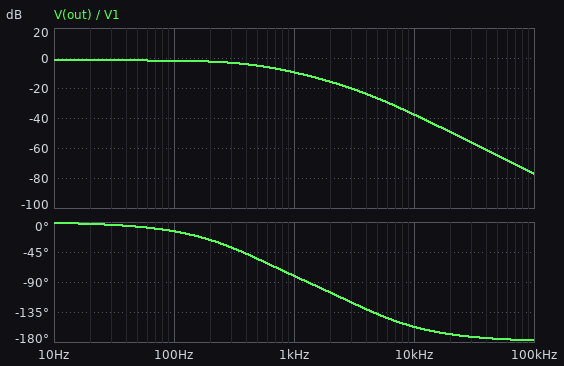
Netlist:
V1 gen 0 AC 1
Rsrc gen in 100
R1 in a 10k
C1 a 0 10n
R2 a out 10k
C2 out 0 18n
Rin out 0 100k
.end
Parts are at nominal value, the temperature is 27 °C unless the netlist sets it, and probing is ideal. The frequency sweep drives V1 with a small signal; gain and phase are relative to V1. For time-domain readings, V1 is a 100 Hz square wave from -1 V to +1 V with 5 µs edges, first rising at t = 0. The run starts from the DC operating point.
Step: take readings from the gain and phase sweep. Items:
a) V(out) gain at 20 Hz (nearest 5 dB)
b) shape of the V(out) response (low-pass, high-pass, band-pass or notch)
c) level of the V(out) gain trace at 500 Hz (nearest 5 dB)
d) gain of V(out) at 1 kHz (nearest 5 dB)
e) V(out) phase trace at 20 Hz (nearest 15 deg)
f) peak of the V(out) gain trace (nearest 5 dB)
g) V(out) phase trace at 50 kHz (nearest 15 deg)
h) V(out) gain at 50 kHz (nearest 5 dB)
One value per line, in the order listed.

0 dB
low-pass
-5 dB
-10 dB
0 deg
0 dB
-180 deg
-65 dB
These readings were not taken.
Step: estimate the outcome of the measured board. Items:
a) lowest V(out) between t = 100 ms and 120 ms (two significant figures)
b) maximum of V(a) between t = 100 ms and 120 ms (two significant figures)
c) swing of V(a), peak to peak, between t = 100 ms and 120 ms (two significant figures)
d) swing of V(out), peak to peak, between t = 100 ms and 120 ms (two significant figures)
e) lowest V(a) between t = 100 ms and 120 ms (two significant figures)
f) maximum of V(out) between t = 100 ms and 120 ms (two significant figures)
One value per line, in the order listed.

-830 mV
920 mV
1.8 V
1.7 V
-920 mV
830 mV
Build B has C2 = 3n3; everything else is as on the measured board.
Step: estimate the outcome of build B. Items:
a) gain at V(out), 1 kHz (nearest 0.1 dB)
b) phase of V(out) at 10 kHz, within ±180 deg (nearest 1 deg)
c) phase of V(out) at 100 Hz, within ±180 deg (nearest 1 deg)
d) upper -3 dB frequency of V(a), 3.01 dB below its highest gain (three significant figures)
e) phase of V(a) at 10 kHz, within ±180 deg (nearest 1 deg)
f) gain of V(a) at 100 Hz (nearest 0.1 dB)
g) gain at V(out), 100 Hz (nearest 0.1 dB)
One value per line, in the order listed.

-3.8 dB
-137 deg
-5 deg
1.30 kHz
-75 deg
-0.8 dB
-1.6 dB
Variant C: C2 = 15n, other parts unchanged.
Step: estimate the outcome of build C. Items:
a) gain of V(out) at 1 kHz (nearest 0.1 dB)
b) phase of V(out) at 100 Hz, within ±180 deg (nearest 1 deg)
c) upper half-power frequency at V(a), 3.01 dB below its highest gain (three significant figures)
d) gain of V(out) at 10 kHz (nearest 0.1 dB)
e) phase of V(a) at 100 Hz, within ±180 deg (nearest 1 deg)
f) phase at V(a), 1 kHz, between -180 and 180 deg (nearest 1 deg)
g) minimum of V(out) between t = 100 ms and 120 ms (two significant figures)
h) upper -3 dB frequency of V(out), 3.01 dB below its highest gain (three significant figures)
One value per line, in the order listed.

-8.5 dB
-12 deg
659 Hz
-36.1 dB
-7 deg
-36 deg
-830 mV
518 Hz
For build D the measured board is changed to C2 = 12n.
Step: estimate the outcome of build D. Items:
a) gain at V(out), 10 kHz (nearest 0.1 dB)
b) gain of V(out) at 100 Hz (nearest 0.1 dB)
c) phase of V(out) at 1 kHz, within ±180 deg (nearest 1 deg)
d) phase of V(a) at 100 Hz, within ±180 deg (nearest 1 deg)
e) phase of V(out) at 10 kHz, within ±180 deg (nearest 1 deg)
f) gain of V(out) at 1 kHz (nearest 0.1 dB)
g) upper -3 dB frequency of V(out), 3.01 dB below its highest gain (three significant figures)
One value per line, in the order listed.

-34.3 dB
-1.7 dB
-72 deg
-7 deg
-155 deg
-7.3 dB
613 Hz
